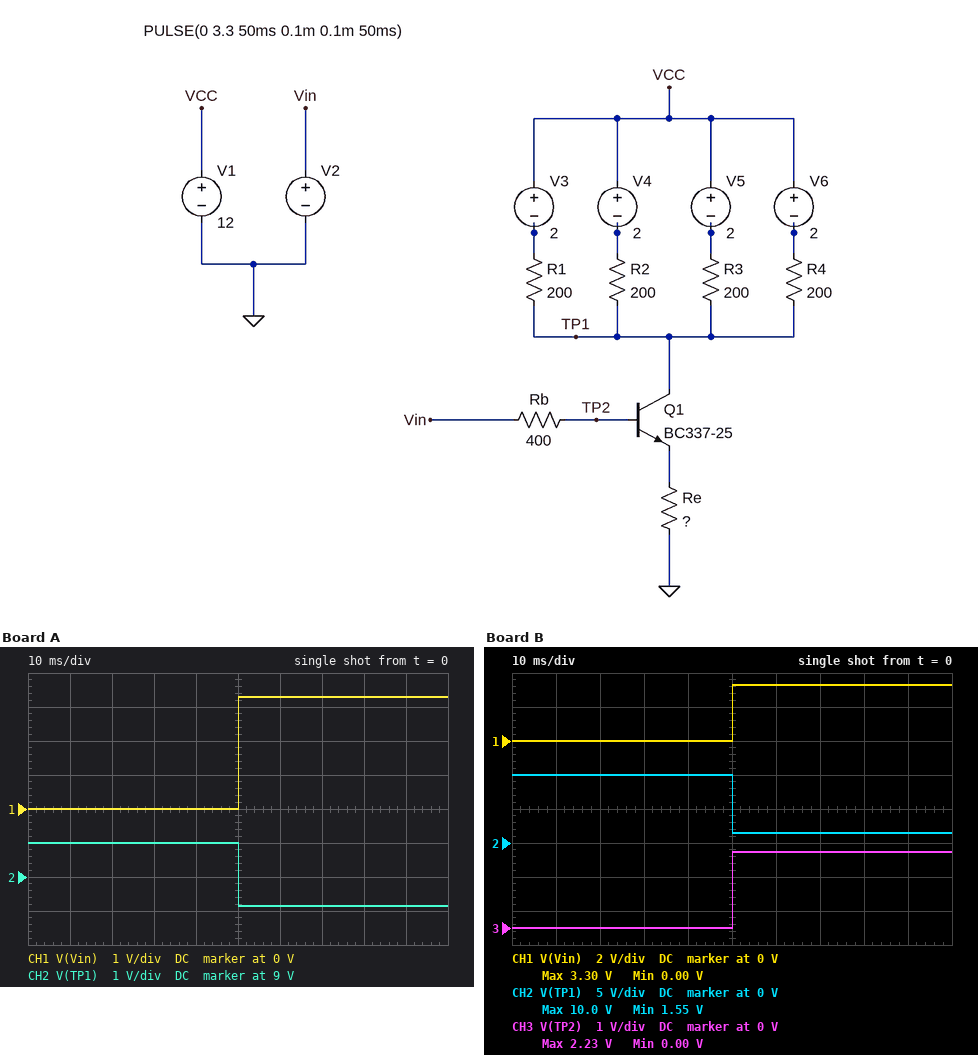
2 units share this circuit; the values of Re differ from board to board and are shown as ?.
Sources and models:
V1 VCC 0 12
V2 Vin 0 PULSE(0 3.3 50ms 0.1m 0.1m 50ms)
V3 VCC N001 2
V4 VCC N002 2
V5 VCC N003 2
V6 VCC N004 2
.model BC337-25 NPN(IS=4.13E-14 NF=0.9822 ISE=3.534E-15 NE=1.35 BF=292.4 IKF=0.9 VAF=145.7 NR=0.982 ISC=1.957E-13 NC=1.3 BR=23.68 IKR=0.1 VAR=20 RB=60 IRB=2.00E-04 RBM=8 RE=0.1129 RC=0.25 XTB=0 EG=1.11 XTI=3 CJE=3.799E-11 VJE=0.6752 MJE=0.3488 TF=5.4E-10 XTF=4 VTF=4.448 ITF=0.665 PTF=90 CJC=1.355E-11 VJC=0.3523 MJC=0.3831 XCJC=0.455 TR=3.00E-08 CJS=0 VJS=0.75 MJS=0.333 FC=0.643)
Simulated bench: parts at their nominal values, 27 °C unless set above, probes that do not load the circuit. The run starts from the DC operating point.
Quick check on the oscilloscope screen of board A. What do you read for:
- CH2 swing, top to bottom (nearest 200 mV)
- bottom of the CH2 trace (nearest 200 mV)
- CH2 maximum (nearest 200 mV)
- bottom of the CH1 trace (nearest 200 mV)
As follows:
1.8 V
8.2 V
10.0 V
0 V
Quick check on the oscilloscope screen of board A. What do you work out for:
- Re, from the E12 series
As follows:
68 Ω
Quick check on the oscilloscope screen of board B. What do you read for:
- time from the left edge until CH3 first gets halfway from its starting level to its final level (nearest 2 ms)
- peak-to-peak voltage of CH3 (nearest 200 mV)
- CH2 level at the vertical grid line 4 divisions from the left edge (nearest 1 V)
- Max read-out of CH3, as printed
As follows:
50 ms
2.2 V
10 V
2.23 V
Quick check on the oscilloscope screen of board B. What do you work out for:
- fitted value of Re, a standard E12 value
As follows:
8.2 Ω
